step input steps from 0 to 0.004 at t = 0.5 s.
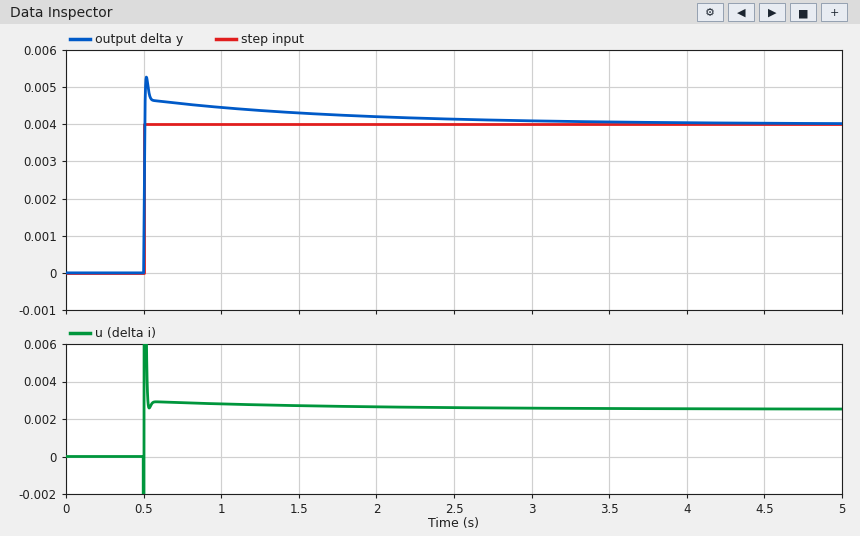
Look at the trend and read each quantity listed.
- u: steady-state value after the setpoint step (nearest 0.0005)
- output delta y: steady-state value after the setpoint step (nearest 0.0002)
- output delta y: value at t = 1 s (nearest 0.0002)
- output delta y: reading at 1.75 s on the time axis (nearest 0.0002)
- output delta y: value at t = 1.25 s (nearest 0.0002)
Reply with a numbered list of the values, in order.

1. 0.0025
2. 0.0040
3. 0.0044
4. 0.0042
5. 0.0044
